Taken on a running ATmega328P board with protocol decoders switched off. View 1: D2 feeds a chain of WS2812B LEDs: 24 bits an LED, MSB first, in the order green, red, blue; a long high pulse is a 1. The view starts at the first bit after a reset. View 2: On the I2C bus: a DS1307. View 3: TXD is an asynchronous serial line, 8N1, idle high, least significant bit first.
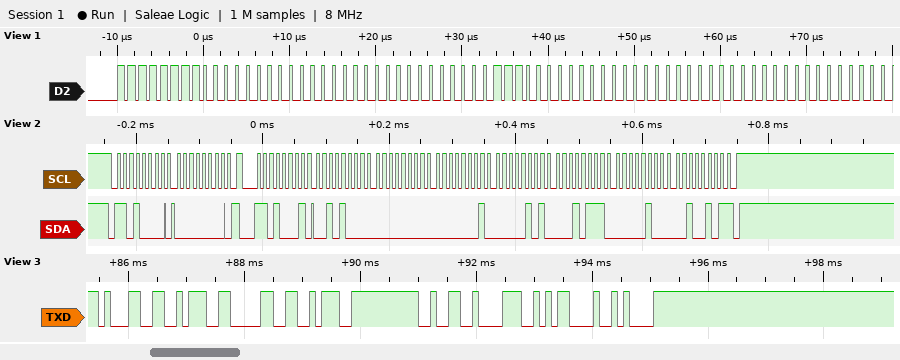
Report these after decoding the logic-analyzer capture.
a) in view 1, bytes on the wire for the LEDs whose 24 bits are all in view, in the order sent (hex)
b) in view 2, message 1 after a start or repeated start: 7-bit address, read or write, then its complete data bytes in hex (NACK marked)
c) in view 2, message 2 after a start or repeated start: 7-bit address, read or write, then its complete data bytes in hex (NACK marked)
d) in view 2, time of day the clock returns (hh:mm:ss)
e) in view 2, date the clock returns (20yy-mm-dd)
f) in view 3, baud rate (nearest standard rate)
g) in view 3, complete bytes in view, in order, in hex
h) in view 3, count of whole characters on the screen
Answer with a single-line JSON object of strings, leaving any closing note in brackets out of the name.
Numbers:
{"in view 1, bytes on the wire for the LEDs whose 24 bits are all in view, in the order sent": "FF 00 00 00 1C 00 00 00 00", "in view 2, message 1 after a start or repeated start: 7-bit address, read or write, then its complete data bytes in hex": "0x68 write: 00", "in view 2, message 2 after a start or repeated start: 7-bit address, read or write, then its complete data bytes in hex": "0x68 read: 28 00 01 05 17 04 25 NACK", "in view 2, time of day the clock returns": "01:00:28", "in view 2, date the clock returns": "2025-04-17", "in view 3, baud rate": "9600 baud", "in view 3, complete bytes in view, in order, in hex": "31 3A 30 3A 32 38 0D 0A", "in view 3, count of whole characters on the screen": "8"}
